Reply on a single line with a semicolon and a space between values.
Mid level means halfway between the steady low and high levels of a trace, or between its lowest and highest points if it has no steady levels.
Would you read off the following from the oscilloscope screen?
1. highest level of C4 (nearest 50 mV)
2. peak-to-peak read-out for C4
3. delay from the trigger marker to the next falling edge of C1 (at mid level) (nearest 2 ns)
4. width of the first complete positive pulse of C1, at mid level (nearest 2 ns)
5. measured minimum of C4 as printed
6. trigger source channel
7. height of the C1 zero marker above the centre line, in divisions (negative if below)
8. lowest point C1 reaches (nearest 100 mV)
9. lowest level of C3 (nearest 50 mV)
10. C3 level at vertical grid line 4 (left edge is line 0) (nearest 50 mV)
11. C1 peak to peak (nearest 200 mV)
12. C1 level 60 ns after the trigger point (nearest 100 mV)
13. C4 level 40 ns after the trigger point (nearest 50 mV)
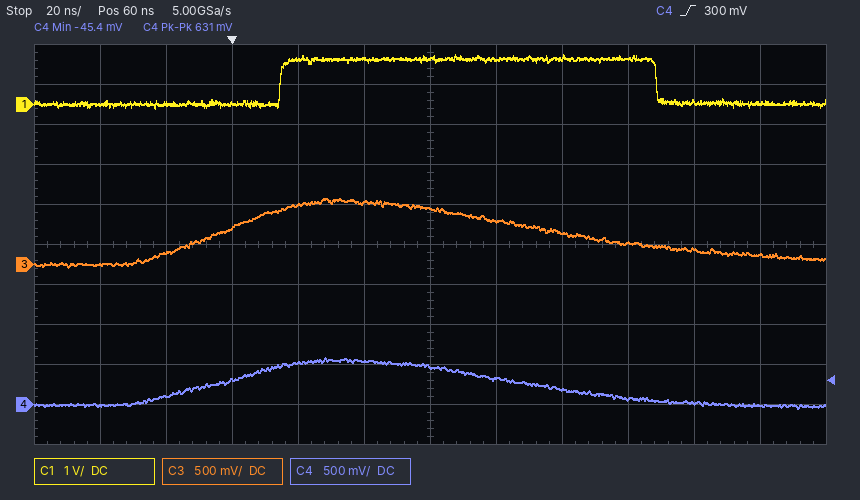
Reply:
600 mV; 631 mV; 128 ns; 114 ns; -45.4 mV; C4; +3.5 div; -100 mV; -50 mV; 750 mV; 1.4 V; 1.1 V; 550 mV
